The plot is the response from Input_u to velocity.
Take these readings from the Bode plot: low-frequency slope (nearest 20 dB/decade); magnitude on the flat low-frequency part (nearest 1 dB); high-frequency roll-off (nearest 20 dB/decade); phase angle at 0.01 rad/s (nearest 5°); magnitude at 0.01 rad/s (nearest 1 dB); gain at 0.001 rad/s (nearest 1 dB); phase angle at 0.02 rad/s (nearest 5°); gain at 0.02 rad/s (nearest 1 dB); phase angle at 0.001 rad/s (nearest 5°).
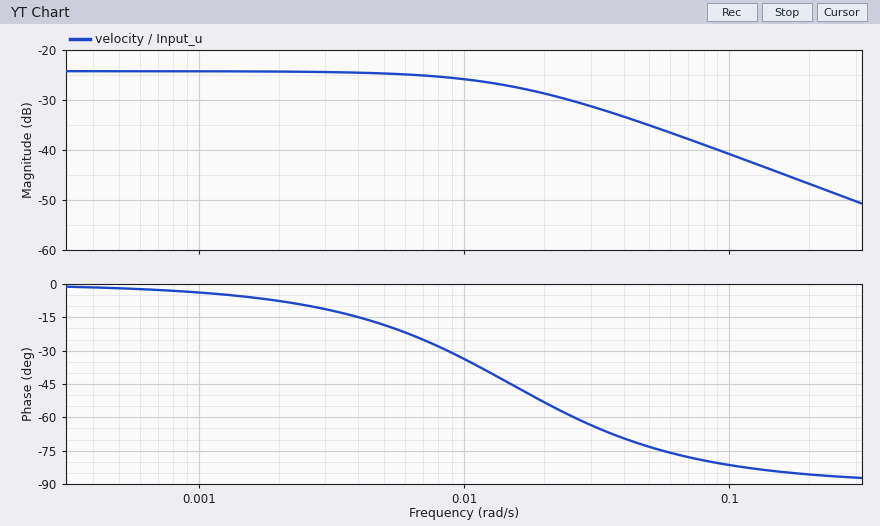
0 dB/decade
-24 dB
-20 dB/decade
-35°
-26 dB
-24 dB
-55°
-29 dB
-5°
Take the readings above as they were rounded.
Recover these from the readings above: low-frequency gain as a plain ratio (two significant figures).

0.063
